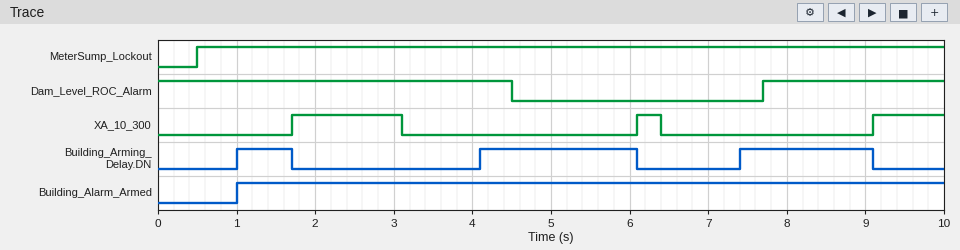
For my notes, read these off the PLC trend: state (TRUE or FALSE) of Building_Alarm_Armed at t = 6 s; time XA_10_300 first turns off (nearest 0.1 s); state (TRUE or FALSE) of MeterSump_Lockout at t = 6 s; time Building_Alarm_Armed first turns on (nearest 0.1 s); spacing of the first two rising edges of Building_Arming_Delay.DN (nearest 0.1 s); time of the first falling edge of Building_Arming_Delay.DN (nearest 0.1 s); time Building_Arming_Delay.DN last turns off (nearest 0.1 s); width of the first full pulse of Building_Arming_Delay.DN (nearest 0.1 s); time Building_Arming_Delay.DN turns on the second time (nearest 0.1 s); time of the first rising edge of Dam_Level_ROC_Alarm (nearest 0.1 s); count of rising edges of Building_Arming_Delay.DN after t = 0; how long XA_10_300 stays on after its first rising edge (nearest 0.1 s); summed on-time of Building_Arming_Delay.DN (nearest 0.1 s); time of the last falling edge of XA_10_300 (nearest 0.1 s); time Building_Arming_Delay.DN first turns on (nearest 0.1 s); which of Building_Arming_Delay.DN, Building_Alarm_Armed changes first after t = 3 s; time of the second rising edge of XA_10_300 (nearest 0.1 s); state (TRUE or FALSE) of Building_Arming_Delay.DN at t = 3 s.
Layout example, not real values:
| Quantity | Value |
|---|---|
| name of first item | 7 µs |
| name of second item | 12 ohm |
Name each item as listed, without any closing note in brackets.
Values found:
| Quantity | Value |
|---|---|
| state (TRUE or FALSE) of Building_Alarm_Armed at t = 6 s | TRUE |
| time XA_10_300 first turns off | 3.1 s |
| state (TRUE or FALSE) of MeterSump_Lockout at t = 6 s | TRUE |
| time Building_Alarm_Armed first turns on | 1.0 s |
| spacing of the first two rising edges of Building_Arming_Delay.DN | 3.1 s |
| time of the first falling edge of Building_Arming_Delay.DN | 1.7 s |
| time Building_Arming_Delay.DN last turns off | 9.1 s |
| width of the first full pulse of Building_Arming_Delay.DN | 0.7 s |
| time Building_Arming_Delay.DN turns on the second time | 4.1 s |
| time of the first rising edge of Dam_Level_ROC_Alarm | 7.7 s |
| count of rising edges of Building_Arming_Delay.DN after t = 0 | 3 |
| how long XA_10_300 stays on after its first rising edge | 1.4 s |
| summed on-time of Building_Arming_Delay.DN | 4.4 s |
| time of the last falling edge of XA_10_300 | 6.4 s |
| time Building_Arming_Delay.DN first turns on | 1.0 s |
| which of Building_Arming_Delay.DN, Building_Alarm_Armed changes first after t = 3 s | Building_Arming_Delay.DN |
| time of the second rising edge of XA_10_300 | 6.1 s |
| state (TRUE or FALSE) of Building_Arming_Delay.DN at t = 3 s | FALSE |
